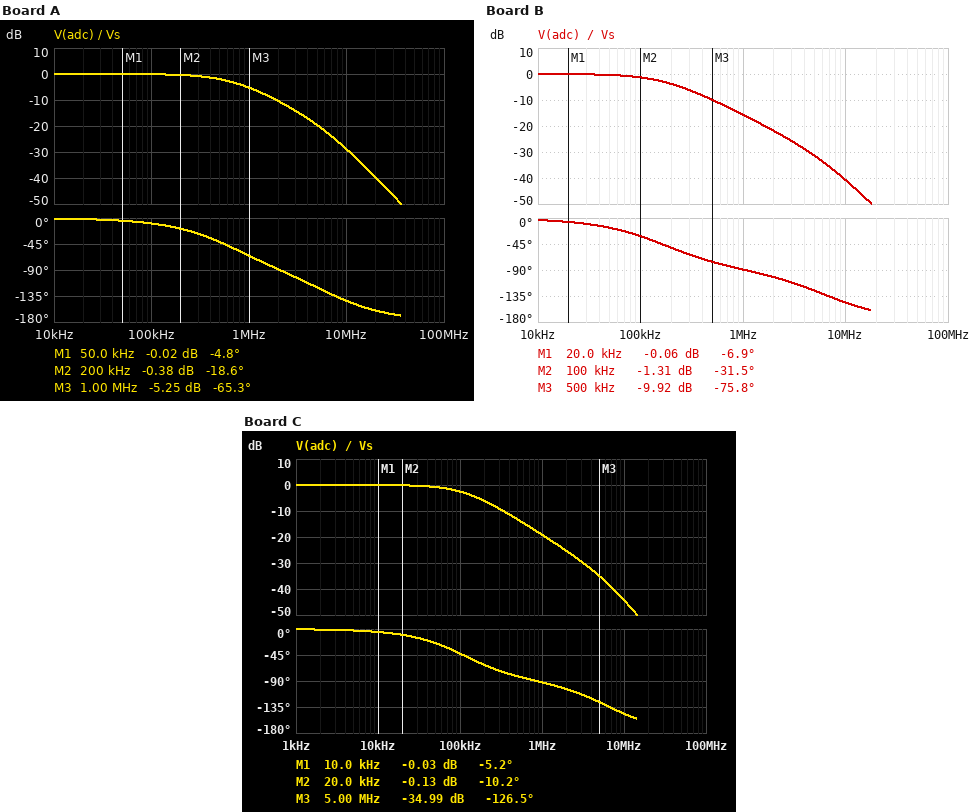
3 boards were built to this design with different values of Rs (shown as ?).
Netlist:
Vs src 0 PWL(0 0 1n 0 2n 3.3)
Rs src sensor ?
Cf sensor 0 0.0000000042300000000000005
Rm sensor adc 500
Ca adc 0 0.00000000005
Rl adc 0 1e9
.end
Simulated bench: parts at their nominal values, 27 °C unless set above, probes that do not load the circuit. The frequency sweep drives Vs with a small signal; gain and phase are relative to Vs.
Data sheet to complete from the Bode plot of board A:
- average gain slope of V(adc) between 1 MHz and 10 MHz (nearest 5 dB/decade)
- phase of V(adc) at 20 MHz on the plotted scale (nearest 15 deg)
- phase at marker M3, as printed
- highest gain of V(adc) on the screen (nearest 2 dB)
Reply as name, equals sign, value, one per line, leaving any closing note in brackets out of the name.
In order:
average gain slope of V(adc) between 1 MHz and 10 MHz = -25 dB/decade
phase of V(adc) at 20 MHz on the plotted scale = -165 deg
phase at marker M3, as printed = -65.3 deg
highest gain of V(adc) on the screen = 0 dB
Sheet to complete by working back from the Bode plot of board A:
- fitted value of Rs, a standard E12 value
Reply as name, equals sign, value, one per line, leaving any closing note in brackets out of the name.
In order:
fitted value of Rs, a standard E12 value = 56 Ω
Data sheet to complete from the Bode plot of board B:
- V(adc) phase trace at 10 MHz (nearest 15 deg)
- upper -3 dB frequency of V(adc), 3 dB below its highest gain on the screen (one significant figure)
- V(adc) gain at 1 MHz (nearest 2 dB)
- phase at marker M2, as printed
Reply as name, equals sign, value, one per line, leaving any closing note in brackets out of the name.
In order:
V(adc) phase trace at 10 MHz = -150 deg
upper -3 dB frequency of V(adc), 3 dB below its highest gain on the screen = 200 kHz
V(adc) gain at 1 MHz = -16 dB
phase at marker M2, as printed = -31.5 deg
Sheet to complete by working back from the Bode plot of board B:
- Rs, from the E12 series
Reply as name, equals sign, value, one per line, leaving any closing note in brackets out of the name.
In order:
Rs, from the E12 series = 220 Ω
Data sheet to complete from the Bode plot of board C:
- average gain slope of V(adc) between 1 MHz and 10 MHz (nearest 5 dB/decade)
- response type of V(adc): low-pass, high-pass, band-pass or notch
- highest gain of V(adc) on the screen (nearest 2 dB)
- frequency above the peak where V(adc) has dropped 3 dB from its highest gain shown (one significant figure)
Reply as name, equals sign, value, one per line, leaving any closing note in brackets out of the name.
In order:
average gain slope of V(adc) between 1 MHz and 10 MHz = -25 dB/decade
response type of V(adc): low-pass, high-pass, band-pass or notch = low-pass
highest gain of V(adc) on the screen = 0 dB
frequency above the peak where V(adc) has dropped 3 dB from its highest gain shown = 100 kHz
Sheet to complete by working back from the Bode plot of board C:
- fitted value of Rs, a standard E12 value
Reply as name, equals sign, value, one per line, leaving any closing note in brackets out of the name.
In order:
fitted value of Rs, a standard E12 value = 330 Ω
